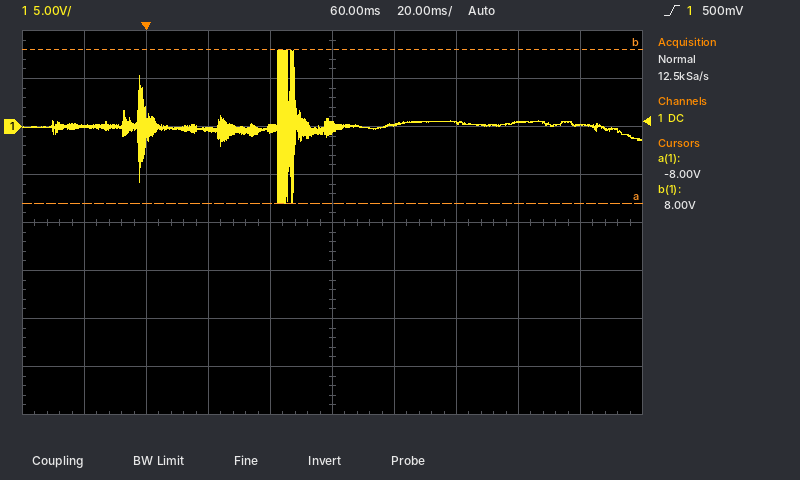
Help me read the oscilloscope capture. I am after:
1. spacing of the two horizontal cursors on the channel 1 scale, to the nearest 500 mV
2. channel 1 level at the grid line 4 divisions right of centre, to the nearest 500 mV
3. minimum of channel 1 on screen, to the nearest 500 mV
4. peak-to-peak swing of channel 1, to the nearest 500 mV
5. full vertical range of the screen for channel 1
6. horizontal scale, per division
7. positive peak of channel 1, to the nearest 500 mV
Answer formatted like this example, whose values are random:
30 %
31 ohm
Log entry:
16.0 V
0.0 V
-8.0 V
16.0 V
40 V
20 ms
8.0 V
